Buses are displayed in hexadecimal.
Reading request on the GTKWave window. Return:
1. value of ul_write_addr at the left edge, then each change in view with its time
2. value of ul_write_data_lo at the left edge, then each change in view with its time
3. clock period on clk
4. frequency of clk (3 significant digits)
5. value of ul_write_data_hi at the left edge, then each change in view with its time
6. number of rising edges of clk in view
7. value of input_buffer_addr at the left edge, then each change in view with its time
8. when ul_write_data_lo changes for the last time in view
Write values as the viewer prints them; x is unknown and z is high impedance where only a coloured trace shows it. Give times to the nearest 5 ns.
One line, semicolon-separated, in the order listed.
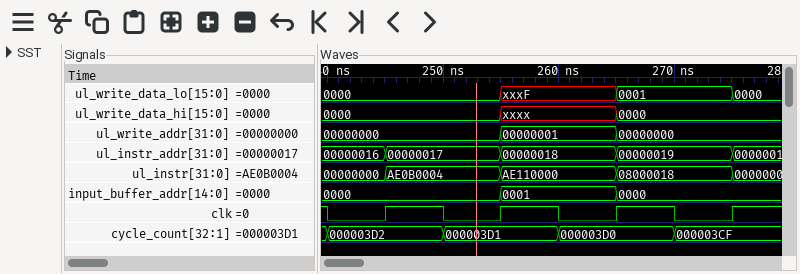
00000000, 00000001 at 255 ns, 00000000 at 265 ns; 0000, xxxF at 255 ns, 0001 at 265 ns, 0000 at 275 ns; 10 ns; 100 MHz; 0000, xxxx at 255 ns, 0000 at 265 ns; 4; 0000, 0001 at 255 ns, 0000 at 265 ns; 275 ns
